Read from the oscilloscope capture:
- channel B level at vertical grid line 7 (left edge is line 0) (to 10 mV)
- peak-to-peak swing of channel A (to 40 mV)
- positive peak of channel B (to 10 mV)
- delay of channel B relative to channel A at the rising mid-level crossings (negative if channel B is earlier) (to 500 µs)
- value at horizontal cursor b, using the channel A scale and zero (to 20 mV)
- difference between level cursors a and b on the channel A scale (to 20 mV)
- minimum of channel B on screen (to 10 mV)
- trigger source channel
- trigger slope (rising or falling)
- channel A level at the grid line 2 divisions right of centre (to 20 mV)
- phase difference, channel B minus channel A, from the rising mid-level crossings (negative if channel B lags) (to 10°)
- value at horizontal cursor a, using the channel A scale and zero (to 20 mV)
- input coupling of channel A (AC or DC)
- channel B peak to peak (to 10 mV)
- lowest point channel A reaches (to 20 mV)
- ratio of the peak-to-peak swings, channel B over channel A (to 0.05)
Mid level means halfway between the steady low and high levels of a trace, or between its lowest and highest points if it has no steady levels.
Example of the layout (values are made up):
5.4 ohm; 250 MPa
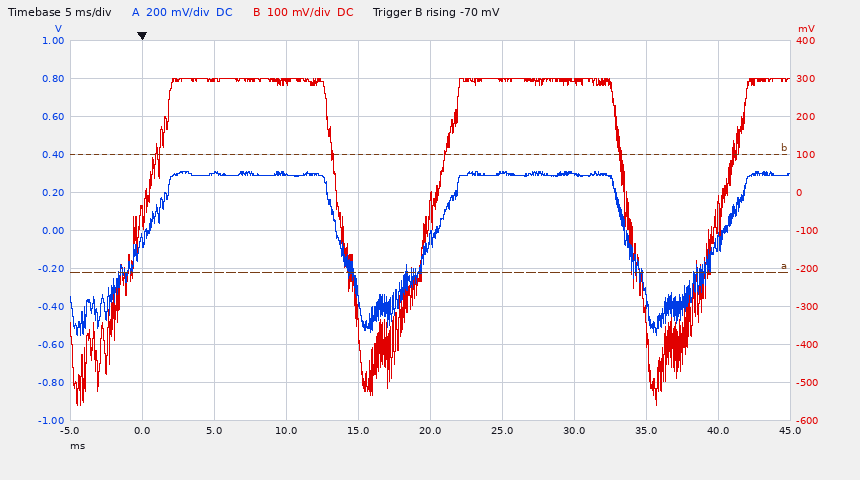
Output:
290 mV; 880 mV; 300 mV; 0.0 ms; 400 mV; 620 mV; -560 mV; channel B; rising; 300 mV; 0°; -220 mV; DC; 860 mV; -560 mV; 1.00
